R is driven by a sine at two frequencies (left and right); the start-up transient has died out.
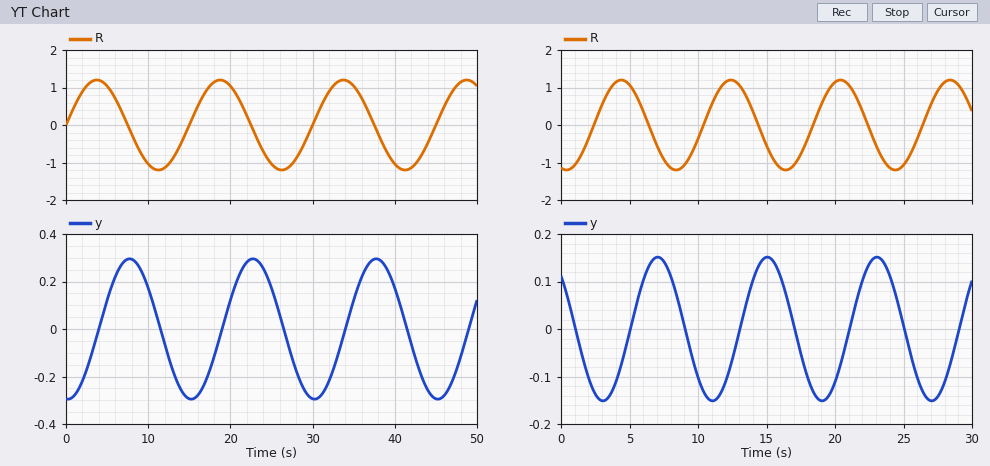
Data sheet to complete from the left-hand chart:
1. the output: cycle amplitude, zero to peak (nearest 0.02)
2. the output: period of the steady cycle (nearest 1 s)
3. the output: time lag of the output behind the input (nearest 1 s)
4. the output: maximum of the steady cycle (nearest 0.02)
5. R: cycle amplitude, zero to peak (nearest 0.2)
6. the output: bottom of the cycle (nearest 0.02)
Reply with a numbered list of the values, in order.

1. 0.30
2. 15 s
3. 4 s
4. 0.30
5. 1.2
6. -0.30
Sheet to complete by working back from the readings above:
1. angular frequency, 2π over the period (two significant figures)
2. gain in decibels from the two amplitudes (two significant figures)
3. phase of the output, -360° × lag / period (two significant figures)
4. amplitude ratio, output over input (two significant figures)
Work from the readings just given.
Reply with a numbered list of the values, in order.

1. 0.42 rad/s
2. -12 dB
3. -96°
4. 0.25
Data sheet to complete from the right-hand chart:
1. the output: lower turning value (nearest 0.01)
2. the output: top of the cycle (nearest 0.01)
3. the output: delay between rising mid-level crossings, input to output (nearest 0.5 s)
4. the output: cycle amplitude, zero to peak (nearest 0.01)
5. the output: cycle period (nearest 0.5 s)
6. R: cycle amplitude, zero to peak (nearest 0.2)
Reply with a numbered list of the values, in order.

1. -0.15
2. 0.15
3. 2.5 s
4. 0.15
5. 8.0 s
6. 1.2
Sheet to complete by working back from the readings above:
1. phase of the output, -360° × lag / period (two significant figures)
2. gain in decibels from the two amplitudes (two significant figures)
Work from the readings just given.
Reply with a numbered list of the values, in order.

1. -110°
2. -18 dB
